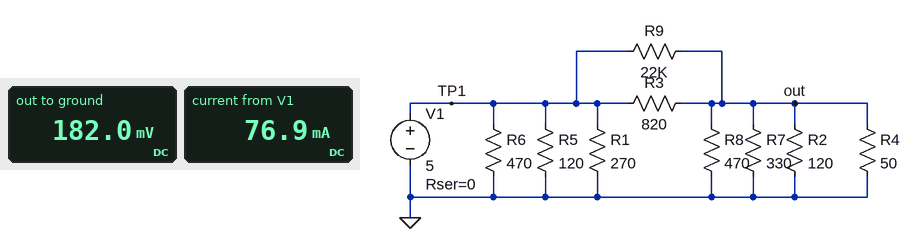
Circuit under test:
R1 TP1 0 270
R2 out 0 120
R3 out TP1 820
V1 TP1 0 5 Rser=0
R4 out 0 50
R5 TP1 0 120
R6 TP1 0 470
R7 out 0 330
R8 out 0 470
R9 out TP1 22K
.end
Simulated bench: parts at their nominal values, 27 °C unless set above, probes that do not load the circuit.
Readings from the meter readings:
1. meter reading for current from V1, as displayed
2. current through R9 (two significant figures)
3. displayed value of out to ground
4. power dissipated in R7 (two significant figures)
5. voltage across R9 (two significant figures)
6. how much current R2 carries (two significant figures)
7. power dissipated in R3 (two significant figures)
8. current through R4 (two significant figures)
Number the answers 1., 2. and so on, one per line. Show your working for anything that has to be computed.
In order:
1. 76.9 mA
2. (5 V - 182 mV) / 22 kΩ = 220 µA
3. 182.0 mV
4. (182 mV)^2 / 330 Ω = 100 µW
5. 5 V - 182 mV = 4.8 V
6. (182 mV) / 120 Ω = 1.5 mA
7. (5 V - 182 mV)^2 / 820 Ω = 28 mW
8. (182 mV) / 50 Ω = 3.6 mA
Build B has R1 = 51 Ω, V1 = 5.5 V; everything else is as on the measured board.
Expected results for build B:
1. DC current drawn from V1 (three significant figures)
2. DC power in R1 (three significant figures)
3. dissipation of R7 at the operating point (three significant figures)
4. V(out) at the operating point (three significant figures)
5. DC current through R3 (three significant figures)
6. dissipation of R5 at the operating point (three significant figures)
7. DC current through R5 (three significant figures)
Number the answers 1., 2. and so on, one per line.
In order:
1. 172 mA
2. 593 mW
3. 121 µW
4. 200 mV
5. 6.46 mA
6. 252 mW
7. 45.8 mA
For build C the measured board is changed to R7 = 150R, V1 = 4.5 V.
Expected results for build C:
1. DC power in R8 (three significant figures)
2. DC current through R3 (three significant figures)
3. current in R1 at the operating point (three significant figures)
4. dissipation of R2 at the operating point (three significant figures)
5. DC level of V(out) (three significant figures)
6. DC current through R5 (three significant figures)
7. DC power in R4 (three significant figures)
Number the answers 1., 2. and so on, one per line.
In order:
1. 46.8 µW
2. 5.31 mA
3. 16.7 mA
4. 183 µW
5. 148 mV
6. 37.5 mA
7. 440 µW
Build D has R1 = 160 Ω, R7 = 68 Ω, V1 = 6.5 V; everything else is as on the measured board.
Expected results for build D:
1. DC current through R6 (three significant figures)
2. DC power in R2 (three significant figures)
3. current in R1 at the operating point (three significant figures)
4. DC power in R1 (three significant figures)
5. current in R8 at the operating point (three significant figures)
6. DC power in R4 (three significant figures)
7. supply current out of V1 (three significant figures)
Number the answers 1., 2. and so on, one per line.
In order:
1. 13.8 mA
2. 261 µW
3. 40.6 mA
4. 264 mW
5. 377 µA
6. 627 µW
7. 117 mA
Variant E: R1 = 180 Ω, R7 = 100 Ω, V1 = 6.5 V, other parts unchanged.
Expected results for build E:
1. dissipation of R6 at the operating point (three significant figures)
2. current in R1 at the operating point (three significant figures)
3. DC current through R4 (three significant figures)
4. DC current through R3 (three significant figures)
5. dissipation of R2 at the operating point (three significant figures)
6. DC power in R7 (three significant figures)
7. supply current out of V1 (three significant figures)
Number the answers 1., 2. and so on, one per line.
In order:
1. 89.9 mW
2. 36.1 mA
3. 3.94 mA
4. 7.69 mA
5. 324 µW
6. 388 µW
7. 112 mA
